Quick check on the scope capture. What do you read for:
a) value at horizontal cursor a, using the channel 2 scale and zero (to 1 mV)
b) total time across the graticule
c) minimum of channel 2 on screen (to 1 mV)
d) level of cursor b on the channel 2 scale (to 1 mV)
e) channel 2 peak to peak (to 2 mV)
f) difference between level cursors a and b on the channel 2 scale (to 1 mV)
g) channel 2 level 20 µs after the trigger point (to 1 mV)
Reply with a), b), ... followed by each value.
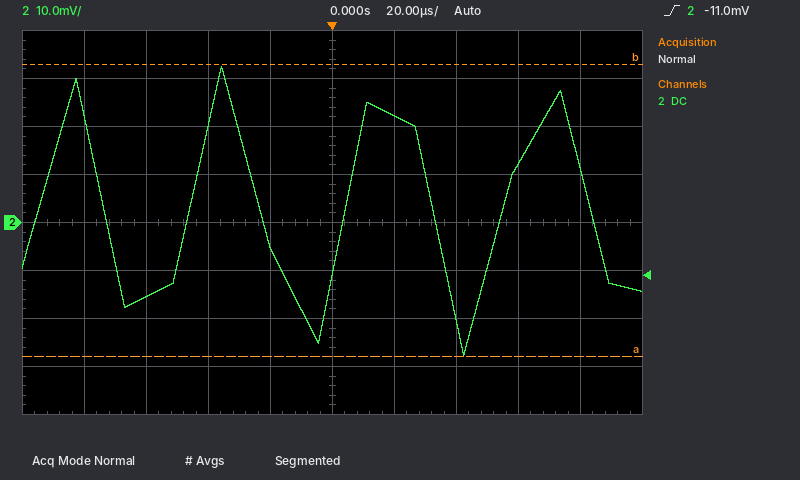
a) -28 mV
b) 200 µs
c) -28 mV
d) 33 mV
e) 60 mV
f) 61 mV
g) 22 mV
